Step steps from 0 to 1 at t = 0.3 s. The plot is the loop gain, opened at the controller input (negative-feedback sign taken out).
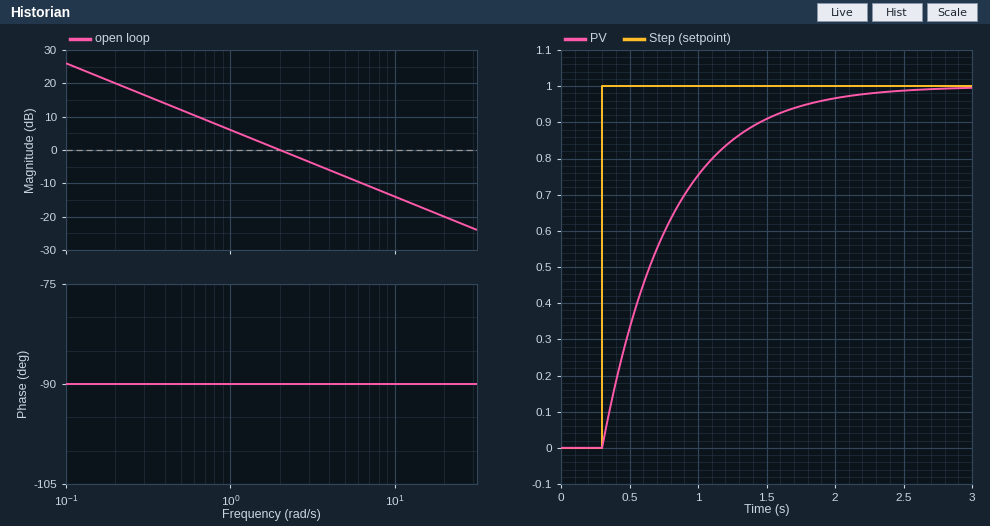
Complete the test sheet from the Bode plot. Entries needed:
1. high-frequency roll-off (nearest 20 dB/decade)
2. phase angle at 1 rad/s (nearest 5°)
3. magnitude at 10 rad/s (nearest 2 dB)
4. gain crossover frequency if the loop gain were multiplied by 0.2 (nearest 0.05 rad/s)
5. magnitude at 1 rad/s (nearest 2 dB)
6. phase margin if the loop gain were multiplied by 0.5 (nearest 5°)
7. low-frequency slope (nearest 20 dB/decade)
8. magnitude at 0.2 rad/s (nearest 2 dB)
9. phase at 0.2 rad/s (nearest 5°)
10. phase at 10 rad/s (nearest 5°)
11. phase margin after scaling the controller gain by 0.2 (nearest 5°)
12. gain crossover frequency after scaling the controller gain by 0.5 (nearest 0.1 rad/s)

-20 dB/decade
-90°
-14 dB
0.40 rad/s
6 dB
90°
-20 dB/decade
20 dB
-90°
-90°
90°
1.0 rad/s
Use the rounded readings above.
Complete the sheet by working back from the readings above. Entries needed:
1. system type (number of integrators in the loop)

1
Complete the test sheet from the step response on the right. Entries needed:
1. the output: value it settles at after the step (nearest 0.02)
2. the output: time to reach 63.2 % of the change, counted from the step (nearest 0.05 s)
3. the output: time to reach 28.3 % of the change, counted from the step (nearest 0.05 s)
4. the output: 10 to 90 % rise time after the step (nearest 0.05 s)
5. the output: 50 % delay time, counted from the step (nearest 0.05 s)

1.00
0.50 s
0.15 s
1.10 s
0.35 s
